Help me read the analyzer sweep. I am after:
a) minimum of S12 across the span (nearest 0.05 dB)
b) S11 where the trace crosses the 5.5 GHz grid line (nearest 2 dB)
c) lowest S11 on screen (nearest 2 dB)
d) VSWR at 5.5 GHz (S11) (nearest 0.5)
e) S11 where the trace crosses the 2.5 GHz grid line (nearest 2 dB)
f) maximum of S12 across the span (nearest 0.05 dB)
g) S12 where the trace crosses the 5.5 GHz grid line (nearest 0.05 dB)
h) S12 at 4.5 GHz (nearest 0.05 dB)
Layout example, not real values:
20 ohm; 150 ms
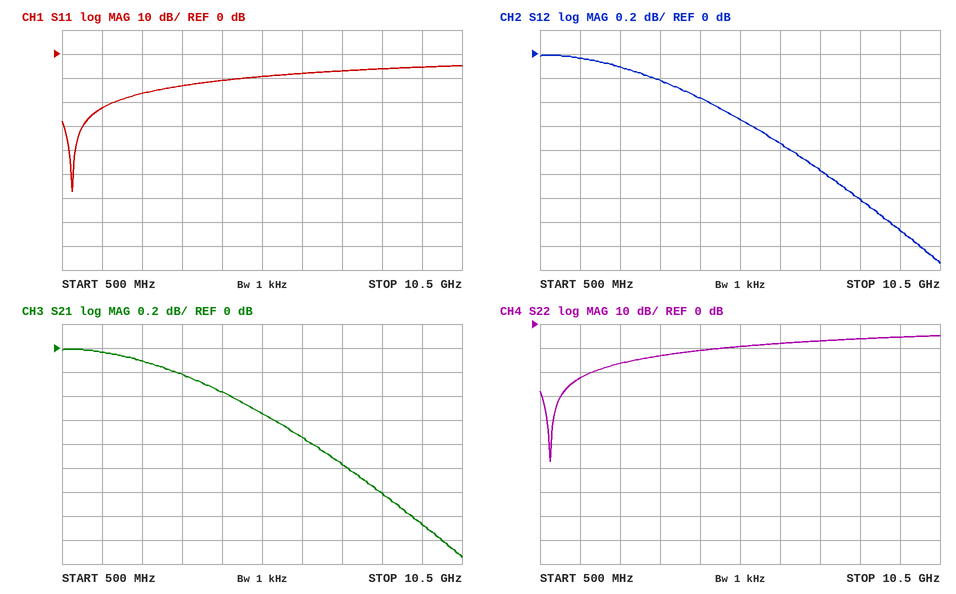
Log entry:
-1.75 dB; -10 dB; -58 dB; 2.0; -16 dB; 0.00 dB; -0.55 dB; -0.35 dB
